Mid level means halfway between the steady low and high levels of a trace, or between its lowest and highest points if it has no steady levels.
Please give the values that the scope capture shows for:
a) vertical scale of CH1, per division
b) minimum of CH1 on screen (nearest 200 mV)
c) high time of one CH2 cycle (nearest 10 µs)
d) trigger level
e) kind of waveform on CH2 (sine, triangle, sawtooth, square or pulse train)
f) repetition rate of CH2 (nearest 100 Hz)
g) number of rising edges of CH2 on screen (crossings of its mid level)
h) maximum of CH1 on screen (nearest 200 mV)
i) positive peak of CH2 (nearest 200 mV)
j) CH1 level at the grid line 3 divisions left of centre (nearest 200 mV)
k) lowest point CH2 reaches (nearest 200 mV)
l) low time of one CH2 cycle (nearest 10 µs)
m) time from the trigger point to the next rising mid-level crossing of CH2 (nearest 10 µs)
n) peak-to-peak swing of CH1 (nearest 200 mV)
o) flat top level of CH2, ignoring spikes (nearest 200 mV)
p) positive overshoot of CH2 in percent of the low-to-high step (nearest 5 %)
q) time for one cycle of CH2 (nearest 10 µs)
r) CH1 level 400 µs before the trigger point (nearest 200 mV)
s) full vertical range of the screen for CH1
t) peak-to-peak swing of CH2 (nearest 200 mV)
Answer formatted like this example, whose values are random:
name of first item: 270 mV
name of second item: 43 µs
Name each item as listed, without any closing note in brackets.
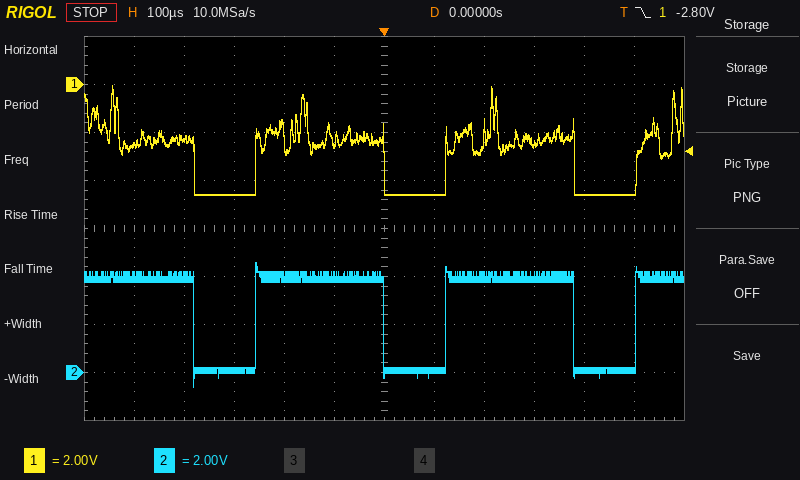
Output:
vertical scale of CH1, per division: 2 V
minimum of CH1 on screen: -4.6 V
high time of one CH2 cycle: 260 µs
trigger level: -2.80 V
kind of waveform on CH2: pulse train
repetition rate of CH2: 2.6 kHz
number of rising edges of CH2 on screen: 3
maximum of CH1 on screen: 0.0 V
positive peak of CH2: 4.6 V
CH1 level at the grid line 3 divisions left of centre: -4.6 V
lowest point CH2 reaches: -600 mV
low time of one CH2 cycle: 120 µs
time from the trigger point to the next rising mid-level crossing of CH2: 120 µs
peak-to-peak swing of CH1: 4.6 V
flat top level of CH2, ignoring spikes: 4.0 V
positive overshoot of CH2 in percent of the low-to-high step: 15 %
time for one cycle of CH2: 380 µs
CH1 level 400 µs before the trigger point: -2.2 V
full vertical range of the screen for CH1: 16 V
peak-to-peak swing of CH2: 5.2 V
